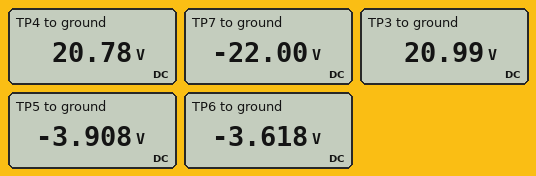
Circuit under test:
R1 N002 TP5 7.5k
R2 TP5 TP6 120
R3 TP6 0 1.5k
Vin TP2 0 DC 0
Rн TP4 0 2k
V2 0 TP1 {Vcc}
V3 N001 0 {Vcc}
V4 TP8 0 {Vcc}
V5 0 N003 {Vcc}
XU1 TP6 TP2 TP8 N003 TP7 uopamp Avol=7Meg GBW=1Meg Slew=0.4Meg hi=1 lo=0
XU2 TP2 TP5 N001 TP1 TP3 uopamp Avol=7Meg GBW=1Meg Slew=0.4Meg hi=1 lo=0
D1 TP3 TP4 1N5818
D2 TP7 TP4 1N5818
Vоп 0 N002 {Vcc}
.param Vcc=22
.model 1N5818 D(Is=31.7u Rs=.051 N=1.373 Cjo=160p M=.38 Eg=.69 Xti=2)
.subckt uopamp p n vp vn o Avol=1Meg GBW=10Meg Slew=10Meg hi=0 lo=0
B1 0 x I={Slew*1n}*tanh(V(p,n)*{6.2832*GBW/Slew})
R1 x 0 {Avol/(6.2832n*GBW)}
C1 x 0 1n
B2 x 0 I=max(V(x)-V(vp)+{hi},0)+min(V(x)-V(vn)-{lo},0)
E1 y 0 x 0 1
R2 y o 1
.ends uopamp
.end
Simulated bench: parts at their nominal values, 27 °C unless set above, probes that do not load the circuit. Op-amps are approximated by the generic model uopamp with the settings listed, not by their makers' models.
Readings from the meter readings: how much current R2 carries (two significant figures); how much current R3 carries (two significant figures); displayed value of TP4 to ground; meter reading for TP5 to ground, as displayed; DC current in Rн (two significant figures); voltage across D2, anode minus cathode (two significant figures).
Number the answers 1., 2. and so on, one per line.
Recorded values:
1. 2.4 mA
2. 2.4 mA
3. 20.78 V
4. -3.908 V
5. 10 mA
6. -43 V
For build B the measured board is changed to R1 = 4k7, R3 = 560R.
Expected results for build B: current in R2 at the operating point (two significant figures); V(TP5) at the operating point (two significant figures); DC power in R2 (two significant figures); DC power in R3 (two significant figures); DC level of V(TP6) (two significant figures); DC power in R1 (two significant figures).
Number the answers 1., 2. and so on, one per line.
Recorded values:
1. 4.1 mA
2. -2.8 V
3. 2.0 mW
4. 9.4 mW
5. -2.3 V
6. 79 mW
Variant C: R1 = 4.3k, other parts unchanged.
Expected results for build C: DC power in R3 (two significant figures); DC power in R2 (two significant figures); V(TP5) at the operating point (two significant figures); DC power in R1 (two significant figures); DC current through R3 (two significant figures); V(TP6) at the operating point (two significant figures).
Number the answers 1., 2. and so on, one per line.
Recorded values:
1. 21 mW
2. 1.7 mW
3. -6.0 V
4. 59 mW
5. 3.7 mA
6. -5.6 V
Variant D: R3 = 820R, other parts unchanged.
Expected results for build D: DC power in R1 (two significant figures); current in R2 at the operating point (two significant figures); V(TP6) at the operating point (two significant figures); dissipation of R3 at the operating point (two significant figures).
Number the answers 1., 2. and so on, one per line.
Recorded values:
1. 51 mW
2. 2.6 mA
3. -2.1 V
4. 5.6 mW
